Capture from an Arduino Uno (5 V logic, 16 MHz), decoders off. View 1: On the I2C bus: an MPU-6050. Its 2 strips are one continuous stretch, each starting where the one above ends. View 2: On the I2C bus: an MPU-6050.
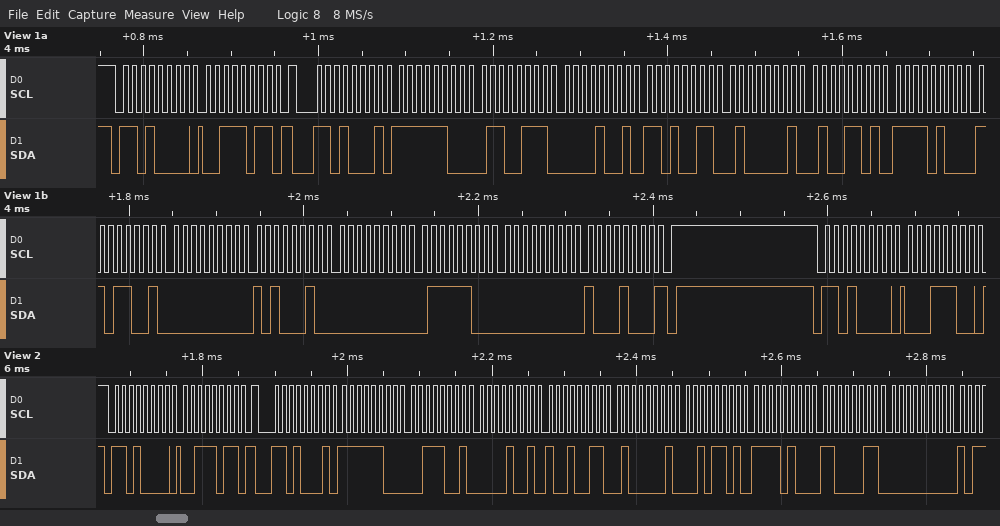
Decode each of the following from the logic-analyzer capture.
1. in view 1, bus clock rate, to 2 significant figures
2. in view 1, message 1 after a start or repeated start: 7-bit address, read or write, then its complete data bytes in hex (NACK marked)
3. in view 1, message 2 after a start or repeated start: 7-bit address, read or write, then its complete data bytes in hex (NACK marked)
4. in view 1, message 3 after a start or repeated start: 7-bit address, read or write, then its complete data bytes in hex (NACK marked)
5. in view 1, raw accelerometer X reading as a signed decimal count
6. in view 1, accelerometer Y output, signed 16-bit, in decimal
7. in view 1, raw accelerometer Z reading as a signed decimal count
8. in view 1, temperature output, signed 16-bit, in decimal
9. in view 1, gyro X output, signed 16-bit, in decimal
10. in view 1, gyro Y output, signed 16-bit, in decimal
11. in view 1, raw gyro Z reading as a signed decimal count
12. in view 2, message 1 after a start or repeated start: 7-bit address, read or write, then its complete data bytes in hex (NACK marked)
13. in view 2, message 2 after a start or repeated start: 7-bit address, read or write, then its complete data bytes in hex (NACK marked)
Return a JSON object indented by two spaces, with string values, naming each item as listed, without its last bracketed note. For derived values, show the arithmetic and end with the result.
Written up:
{
  "in view 1, bus clock rate, to 2 significant figures": "100 kHz",
  "in view 1, message 1 after a start or repeated start: 7-bit address, read or write, then its complete data bytes in hex": "0x68 write: 3B",
  "in view 1, message 2 after a start or repeated start: 7-bit address, read or write, then its complete data bytes in hex": "0x68 read: FC 67 09 D3 41 4D F4 D9 00 A2 00 7C 00 88 NACK",
  "in view 1, message 3 after a start or repeated start: 7-bit address, read or write, then its complete data bytes in hex": "0x68 write: 1C",
  "in view 1, raw accelerometer X reading as a signed decimal count": "0xFC67 = -921",
  "in view 1, accelerometer Y output, signed 16-bit, in decimal": "0x09D3 = 2515",
  "in view 1, raw accelerometer Z reading as a signed decimal count": "0x414D = 16717",
  "in view 1, temperature output, signed 16-bit, in decimal": "0xF4D9 = -2855",
  "in view 1, gyro X output, signed 16-bit, in decimal": "0x00A2 = 162",
  "in view 1, gyro Y output, signed 16-bit, in decimal": "0x007C = 124",
  "in view 1, raw gyro Z reading as a signed decimal count": "0x0088 = 136",
  "in view 2, message 1 after a start or repeated start: 7-bit address, read or write, then its complete data bytes in hex": "0x68 write: 3B",
  "in view 2, message 2 after a start or repeated start: 7-bit address, read or write, then its complete data bytes in hex": "0x68 read: FC 39 09 93 41 2D F4 C3 00"
}
